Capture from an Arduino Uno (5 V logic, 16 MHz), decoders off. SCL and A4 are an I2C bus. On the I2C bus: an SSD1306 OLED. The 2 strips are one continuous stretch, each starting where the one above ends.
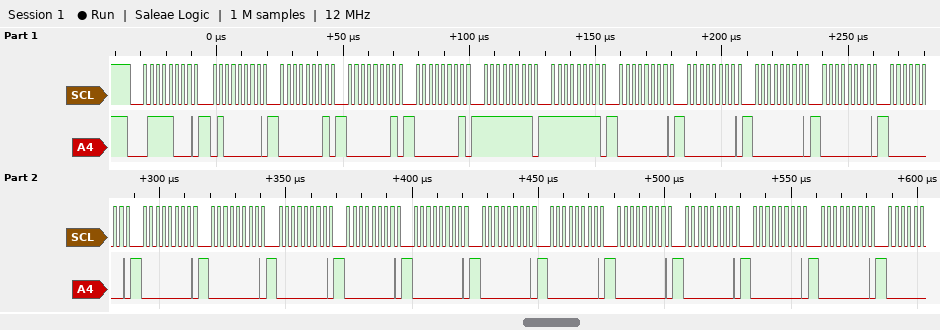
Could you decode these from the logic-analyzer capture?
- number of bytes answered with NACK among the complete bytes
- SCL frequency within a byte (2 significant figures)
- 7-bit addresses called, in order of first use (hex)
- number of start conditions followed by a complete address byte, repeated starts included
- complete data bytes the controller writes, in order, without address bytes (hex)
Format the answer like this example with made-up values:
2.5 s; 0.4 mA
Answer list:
0; 400 kHz; 0x3C; 1; 40 01 01 01 FF FF 00 00 00 00 00 00 00 00 00 00 00 00 00 00 00 00
